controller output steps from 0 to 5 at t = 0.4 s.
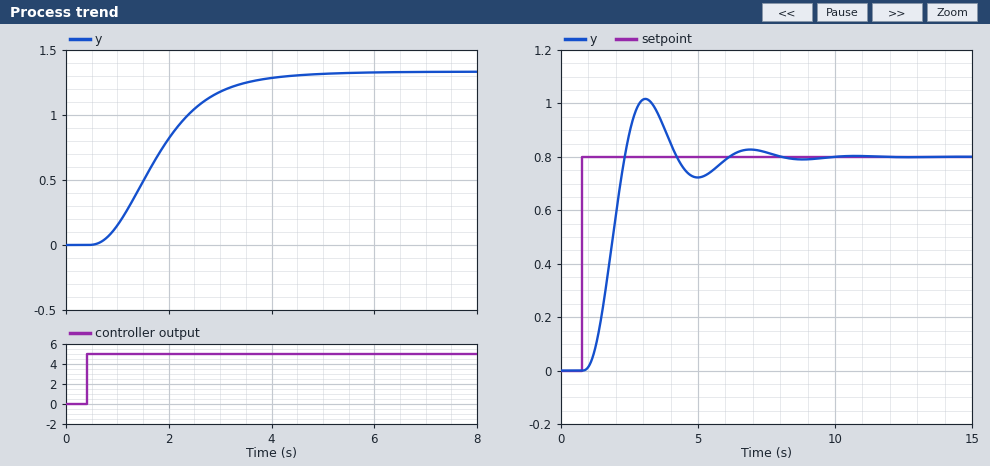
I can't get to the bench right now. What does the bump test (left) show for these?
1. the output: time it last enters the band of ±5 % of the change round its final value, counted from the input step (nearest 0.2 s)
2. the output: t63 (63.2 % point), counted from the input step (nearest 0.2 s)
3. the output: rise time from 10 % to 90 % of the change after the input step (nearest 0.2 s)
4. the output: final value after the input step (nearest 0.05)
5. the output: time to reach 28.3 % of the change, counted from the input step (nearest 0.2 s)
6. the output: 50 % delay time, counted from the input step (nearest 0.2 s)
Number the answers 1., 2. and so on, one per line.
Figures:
1. 3.4 s
2. 1.6 s
3. 2.2 s
4. 1.35
5. 1.0 s
6. 1.4 s
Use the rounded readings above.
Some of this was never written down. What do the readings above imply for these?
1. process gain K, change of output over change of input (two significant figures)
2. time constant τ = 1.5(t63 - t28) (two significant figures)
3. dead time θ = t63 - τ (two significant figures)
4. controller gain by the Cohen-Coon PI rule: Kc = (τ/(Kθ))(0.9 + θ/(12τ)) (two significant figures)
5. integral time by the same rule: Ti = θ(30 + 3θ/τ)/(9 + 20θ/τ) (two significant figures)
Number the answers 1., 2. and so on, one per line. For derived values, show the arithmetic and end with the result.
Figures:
1. (1.35 - 0) / 5 = 0.27
2. 1.5 × (1.6 - 1) = 0.90 s
3. 1.6 - 0.9 = 0.70 s
4. 0.9 / (0.27 × 0.7) × (0.9 + 0.7 / (12 × 0.9)) = 4.6
5. 0.7 × (30 + 3 × 0.7 / 0.9) / (9 + 20 × 0.7 / 0.9) = 0.92 s
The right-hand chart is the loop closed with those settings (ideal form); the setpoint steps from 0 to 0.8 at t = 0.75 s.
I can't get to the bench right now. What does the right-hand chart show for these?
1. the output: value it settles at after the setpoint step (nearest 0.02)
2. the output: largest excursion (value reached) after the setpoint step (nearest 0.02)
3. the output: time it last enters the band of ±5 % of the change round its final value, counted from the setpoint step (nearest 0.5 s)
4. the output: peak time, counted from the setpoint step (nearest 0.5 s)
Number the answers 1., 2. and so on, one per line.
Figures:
1. 0.80
2. 1.02
3. 5.0 s
4. 2.5 s
